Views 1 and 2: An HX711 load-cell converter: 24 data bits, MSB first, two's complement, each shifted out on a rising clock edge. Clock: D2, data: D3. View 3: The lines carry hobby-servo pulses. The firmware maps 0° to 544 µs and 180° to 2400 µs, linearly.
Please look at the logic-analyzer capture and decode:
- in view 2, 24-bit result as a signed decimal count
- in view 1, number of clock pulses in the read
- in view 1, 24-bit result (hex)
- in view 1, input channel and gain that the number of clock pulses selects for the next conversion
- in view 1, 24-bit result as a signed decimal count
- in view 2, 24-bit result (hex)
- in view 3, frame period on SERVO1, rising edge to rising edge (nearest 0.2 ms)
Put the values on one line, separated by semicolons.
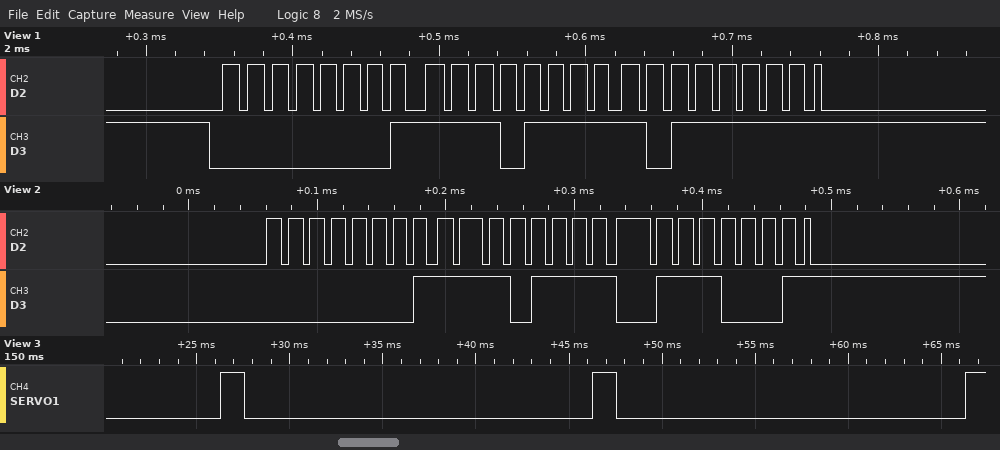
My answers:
126833; 25; 0x01EFBF; channel A, gain 128; 126911; 0x01EF71; 20.0 ms
